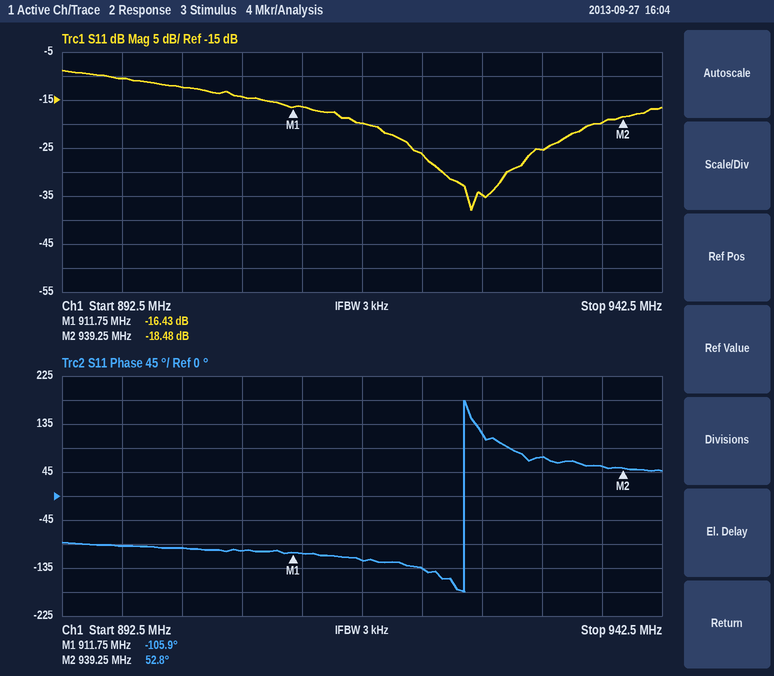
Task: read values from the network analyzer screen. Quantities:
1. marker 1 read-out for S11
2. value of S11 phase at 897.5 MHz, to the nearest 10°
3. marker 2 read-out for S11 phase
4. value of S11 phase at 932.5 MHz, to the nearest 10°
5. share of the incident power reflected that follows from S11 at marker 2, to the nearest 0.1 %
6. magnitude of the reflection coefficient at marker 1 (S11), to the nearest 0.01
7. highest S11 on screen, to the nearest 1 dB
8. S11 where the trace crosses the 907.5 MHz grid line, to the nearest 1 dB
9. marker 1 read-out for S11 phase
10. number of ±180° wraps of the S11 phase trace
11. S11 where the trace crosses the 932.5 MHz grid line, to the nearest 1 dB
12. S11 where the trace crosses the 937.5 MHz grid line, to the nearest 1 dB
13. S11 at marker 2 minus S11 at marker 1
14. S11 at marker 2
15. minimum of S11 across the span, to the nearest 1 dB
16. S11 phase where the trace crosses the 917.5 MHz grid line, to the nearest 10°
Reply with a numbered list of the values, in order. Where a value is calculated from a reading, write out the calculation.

1. -16.43 dB
2. -90°
3. 52.8°
4. 70°
5. 10^(-18.48/10) ≈ 1.4 %
6. 10^(-16.43/20) ≈ 0.15
7. -9 dB
8. -14 dB
9. -105.9°
10. 1
11. -25 dB
12. -20 dB
13. -18.48 − (-16.43) = -2.05 dB
14. -18.48 dB
15. -38 dB
16. -120°
